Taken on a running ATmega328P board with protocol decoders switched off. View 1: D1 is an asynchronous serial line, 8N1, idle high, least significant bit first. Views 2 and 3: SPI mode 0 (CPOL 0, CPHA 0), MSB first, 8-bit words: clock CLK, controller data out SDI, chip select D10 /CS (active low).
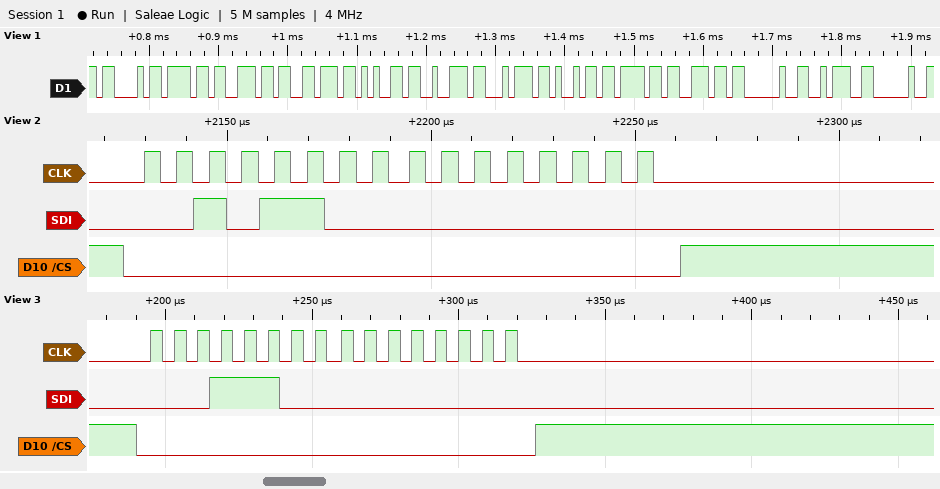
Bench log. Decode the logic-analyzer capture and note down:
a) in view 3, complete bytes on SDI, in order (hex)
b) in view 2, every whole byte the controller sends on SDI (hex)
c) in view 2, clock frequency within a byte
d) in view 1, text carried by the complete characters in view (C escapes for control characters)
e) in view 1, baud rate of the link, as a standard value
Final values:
1C 00
2C 00
125 kHz
"Convertion : "
115200 baud
